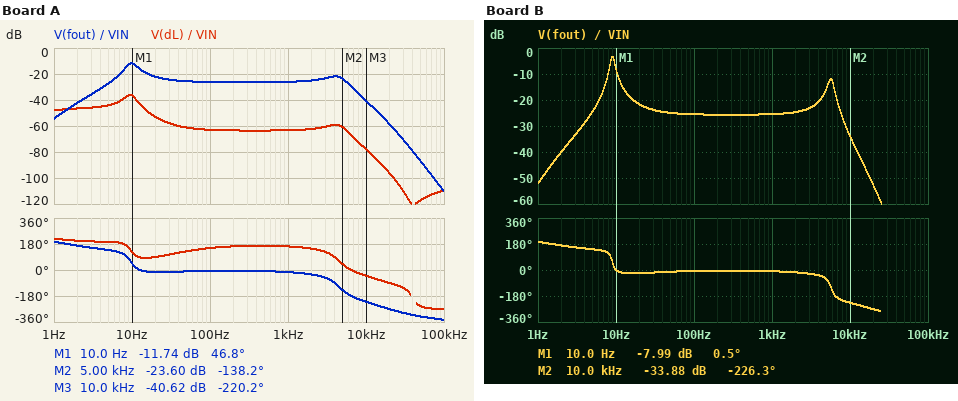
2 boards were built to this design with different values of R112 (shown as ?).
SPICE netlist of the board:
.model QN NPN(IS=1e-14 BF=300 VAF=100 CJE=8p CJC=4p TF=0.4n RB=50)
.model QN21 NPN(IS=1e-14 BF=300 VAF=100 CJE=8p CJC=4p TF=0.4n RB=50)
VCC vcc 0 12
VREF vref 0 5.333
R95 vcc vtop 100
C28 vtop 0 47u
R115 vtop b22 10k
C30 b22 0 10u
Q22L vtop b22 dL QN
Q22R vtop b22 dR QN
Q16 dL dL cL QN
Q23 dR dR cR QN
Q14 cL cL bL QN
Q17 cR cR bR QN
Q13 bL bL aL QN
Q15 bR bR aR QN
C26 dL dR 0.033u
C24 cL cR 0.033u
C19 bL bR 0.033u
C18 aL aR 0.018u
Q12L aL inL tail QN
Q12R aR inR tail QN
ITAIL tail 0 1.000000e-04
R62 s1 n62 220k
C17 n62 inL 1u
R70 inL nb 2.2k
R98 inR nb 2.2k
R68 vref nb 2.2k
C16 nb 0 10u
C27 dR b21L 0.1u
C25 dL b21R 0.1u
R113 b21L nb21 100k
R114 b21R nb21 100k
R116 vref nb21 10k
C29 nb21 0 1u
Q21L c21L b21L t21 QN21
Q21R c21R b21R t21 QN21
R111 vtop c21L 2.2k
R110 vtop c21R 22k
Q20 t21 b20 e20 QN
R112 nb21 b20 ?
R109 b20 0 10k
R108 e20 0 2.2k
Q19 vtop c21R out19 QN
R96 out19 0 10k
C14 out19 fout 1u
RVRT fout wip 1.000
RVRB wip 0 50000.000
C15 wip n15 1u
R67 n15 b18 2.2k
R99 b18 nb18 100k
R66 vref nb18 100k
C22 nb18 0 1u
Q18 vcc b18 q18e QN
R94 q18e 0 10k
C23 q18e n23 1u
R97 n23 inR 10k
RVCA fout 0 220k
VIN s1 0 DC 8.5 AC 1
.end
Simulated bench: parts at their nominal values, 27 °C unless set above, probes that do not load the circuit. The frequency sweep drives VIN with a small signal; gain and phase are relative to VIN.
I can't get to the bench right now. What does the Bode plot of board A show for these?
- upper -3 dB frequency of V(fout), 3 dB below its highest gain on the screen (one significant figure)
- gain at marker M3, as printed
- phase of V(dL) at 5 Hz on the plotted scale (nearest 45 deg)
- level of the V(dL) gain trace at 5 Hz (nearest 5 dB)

10 Hz
-40.62 dB
180 deg
-45 dB
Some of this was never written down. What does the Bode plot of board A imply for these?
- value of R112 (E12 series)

33 kΩ
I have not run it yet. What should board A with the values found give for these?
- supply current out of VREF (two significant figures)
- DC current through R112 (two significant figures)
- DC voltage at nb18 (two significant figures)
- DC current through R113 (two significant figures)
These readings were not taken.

100 µA
100 µA
5.2 V
280 nA
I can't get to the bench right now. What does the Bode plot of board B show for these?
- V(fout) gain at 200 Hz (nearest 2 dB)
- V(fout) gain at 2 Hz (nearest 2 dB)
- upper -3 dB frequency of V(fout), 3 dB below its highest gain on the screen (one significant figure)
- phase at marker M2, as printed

-26 dB
-40 dB
10 Hz
-226.3 deg
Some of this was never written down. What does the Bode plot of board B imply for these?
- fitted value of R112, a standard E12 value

18 kΩ
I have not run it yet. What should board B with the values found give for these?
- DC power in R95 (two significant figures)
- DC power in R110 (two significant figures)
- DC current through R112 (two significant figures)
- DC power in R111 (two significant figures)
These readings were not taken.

140 µW
650 µW
140 µA
68 µW
